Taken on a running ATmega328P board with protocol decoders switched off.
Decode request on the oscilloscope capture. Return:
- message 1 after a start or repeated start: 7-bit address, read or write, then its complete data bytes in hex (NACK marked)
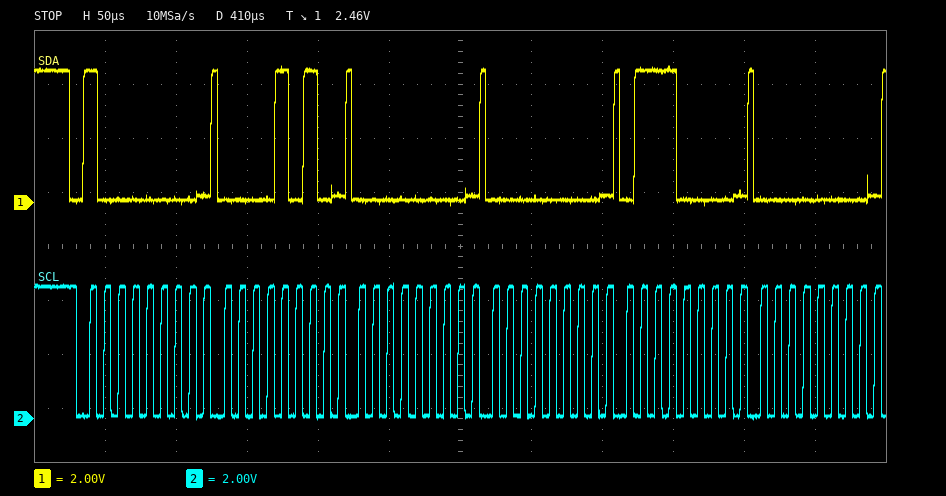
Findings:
0x40 write: 0A 00 00 70 00
